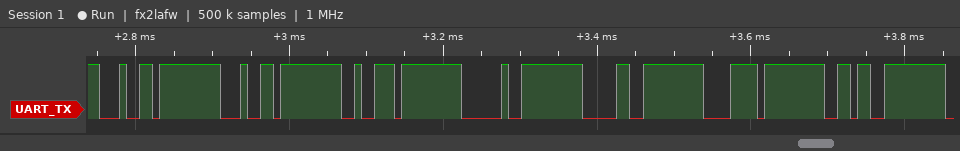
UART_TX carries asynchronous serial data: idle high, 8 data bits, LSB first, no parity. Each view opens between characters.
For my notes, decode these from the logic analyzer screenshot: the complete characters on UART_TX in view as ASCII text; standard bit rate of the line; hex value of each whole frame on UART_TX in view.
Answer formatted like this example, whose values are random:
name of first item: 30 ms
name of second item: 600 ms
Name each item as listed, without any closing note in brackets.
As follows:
the complete characters on UART_TX in view as ASCII text: "ddr 0x6"
standard bit rate of the line: 115200 baud
hex value of each whole frame on UART_TX in view: 64, 64, 72, 20, 30, 78, 36
